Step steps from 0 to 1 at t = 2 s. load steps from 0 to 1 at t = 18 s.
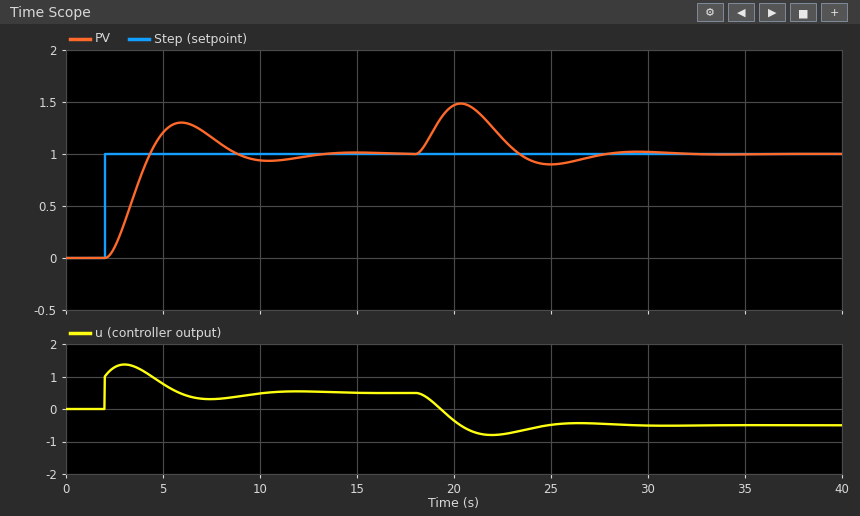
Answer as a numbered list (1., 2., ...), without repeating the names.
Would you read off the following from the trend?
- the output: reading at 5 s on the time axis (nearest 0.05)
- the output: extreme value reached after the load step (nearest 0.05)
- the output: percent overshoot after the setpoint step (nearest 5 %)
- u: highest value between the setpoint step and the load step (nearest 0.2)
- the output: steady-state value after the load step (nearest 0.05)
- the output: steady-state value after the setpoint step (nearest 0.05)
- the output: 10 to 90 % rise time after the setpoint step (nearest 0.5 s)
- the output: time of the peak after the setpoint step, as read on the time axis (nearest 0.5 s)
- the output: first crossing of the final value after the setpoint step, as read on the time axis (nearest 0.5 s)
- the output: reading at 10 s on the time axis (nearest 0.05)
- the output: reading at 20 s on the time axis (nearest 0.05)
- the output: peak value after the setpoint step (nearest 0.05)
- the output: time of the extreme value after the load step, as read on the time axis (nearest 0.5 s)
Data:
1. 1.20
2. 1.50
3. 30 %
4. 1.4
5. 1.00
6. 1.00
7. 1.5 s
8. 6.0 s
9. 4.5 s
10. 0.95
11. 1.45
12. 1.30
13. 20.5 s
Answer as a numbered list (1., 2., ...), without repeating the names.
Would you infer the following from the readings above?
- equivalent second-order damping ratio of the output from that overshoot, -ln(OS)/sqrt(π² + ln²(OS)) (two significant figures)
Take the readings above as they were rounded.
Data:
1. 0.36
